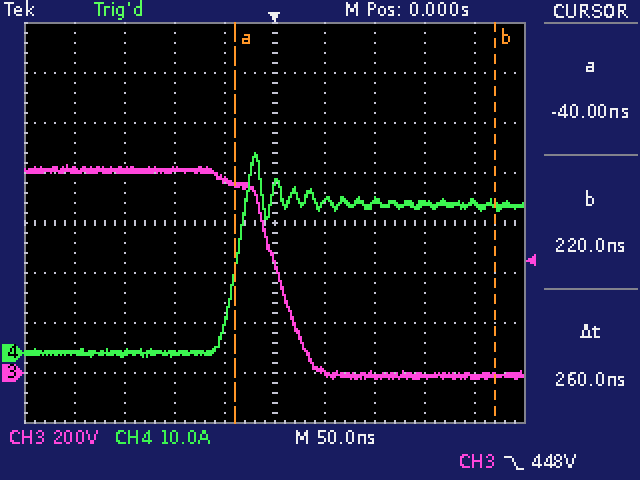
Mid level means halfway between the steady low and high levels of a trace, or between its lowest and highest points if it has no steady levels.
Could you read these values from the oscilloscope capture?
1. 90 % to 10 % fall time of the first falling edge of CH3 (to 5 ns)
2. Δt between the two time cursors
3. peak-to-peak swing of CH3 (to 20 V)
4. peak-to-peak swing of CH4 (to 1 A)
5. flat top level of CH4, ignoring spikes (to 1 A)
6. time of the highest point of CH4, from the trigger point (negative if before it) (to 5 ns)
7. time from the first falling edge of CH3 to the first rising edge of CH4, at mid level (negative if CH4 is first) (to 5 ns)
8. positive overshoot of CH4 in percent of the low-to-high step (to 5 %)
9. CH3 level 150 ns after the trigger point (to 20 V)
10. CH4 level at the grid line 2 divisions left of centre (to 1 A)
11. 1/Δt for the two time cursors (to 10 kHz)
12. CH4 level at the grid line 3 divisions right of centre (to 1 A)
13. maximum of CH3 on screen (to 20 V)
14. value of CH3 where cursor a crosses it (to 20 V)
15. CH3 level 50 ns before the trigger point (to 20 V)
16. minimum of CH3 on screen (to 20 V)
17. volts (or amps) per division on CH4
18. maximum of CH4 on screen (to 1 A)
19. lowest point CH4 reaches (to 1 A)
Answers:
55 ns
260 ns
860 V
41 A
30 A
-20 ns
-45 ns
35 %
-20 V
0 A
3.85 MHz
30 A
840 V
760 V
780 V
-20 V
10 A
40 A
-1 A
